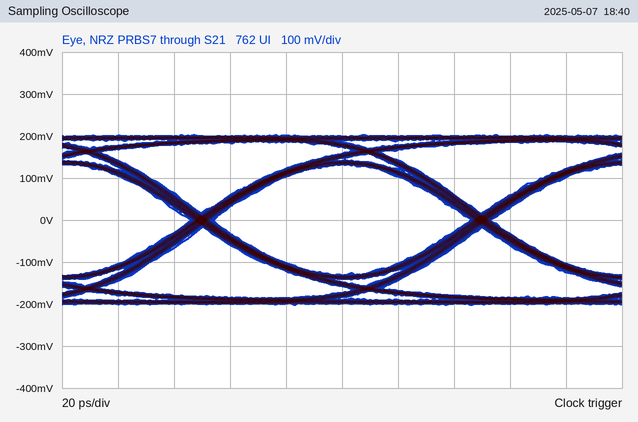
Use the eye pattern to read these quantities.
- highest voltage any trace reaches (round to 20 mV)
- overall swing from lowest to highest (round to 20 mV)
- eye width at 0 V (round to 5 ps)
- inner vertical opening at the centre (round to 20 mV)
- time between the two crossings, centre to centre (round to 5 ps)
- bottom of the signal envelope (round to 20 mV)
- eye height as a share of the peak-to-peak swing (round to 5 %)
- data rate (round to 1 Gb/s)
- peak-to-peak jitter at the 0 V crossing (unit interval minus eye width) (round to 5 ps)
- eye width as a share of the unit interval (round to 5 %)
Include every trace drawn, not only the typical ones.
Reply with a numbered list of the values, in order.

1. 200 mV
2. 400 mV
3. 90 ps
4. 260 mV
5. 100 ps
6. -200 mV
7. 65 %
8. 10 Gb/s
9. 10 ps
10. 90 %
